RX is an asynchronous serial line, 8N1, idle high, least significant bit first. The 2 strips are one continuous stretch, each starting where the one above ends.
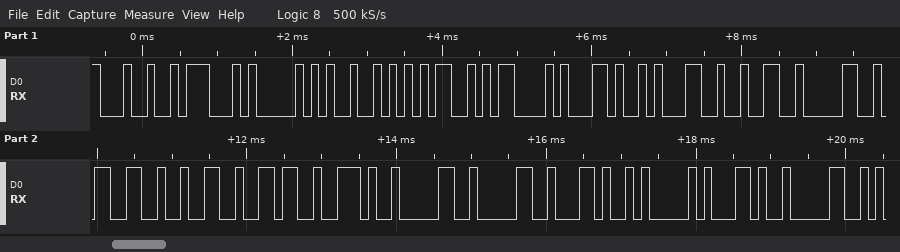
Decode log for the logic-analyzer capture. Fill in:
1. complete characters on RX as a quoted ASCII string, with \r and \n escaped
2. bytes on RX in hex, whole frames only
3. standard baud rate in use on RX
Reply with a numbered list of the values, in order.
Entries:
1. "$GPRMC,120326.00,A,0"
2. 24 47 50 52 4D 43 2C 31 32 30 33 32 36 2E 30 30 2C 41 2C 30
3. 9600 baud
